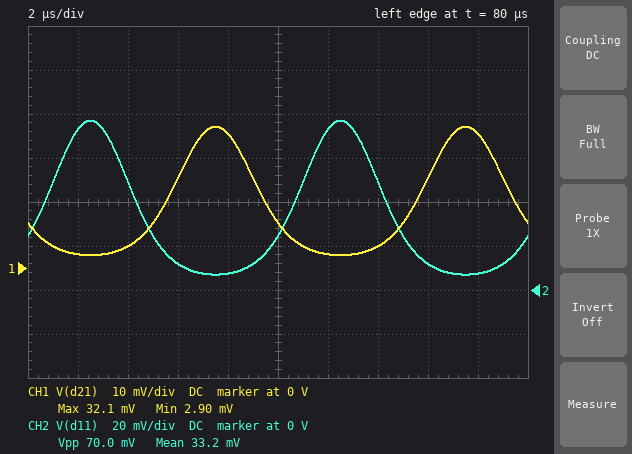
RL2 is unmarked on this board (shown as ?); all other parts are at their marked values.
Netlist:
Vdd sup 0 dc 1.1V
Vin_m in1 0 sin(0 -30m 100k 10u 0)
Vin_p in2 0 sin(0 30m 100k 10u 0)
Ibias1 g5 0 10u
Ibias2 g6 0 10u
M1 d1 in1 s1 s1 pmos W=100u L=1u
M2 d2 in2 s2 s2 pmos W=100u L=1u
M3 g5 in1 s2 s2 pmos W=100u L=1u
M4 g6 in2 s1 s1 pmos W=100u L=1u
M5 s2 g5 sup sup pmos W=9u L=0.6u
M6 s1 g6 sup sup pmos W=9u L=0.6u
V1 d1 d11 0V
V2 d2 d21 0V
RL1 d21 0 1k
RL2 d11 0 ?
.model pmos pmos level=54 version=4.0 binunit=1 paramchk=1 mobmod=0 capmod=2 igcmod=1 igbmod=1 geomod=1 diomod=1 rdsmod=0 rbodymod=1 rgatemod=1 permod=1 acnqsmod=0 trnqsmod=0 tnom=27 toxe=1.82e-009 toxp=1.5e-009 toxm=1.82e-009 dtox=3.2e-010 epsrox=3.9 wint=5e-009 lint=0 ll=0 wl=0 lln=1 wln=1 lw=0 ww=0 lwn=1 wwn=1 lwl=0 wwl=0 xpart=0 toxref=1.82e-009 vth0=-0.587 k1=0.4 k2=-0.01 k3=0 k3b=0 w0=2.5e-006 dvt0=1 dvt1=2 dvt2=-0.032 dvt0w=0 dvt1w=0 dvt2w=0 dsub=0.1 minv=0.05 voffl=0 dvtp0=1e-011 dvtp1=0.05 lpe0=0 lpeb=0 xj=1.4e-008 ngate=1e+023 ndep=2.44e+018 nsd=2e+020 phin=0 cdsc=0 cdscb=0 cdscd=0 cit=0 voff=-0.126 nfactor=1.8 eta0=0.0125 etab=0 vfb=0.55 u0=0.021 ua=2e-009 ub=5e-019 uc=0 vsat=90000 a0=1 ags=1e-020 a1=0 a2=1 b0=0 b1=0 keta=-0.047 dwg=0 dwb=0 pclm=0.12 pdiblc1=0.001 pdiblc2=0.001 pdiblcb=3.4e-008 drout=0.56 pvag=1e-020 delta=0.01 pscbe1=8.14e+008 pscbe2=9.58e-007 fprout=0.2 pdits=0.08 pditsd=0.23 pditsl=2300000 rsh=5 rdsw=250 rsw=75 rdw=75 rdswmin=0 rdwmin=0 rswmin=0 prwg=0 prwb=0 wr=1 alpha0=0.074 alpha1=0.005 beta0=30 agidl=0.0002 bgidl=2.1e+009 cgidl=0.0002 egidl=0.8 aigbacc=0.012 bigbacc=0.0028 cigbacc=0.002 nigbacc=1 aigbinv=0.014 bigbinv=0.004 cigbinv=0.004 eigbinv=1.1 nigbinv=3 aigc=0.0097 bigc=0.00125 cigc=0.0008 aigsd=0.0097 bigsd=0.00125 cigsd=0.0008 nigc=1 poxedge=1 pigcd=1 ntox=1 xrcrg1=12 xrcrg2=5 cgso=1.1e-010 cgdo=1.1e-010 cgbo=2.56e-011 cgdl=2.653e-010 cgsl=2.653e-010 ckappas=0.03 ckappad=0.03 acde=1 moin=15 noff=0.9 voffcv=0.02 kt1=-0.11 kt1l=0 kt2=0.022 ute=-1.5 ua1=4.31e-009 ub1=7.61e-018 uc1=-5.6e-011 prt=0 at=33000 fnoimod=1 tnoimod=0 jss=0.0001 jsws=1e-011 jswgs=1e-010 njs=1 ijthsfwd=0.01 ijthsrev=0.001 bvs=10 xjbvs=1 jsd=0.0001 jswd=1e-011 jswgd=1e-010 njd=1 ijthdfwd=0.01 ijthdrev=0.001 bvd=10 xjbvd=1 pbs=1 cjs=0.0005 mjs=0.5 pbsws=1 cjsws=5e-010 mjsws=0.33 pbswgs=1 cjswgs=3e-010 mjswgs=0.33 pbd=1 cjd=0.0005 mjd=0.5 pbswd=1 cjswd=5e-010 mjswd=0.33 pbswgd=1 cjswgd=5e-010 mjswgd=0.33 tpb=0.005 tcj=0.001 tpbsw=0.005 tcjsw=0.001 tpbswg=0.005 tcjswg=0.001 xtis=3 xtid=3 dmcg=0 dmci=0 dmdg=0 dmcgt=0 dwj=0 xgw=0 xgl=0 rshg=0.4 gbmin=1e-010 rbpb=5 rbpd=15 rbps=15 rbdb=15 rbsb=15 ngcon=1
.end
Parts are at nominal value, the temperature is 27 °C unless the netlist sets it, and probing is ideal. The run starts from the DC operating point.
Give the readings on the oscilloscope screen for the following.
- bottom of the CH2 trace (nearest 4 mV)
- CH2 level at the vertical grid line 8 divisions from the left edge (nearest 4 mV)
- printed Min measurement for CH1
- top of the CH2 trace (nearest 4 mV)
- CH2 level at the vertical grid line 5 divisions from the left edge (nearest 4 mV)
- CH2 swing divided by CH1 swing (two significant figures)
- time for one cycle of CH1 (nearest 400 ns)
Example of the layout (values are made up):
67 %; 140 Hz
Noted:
8 mV; 12 mV; 2.90 mV; 76 mV; 24 mV; 2.4; 10.0 µs
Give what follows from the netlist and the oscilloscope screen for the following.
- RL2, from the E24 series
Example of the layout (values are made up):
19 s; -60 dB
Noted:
2.4 kΩ
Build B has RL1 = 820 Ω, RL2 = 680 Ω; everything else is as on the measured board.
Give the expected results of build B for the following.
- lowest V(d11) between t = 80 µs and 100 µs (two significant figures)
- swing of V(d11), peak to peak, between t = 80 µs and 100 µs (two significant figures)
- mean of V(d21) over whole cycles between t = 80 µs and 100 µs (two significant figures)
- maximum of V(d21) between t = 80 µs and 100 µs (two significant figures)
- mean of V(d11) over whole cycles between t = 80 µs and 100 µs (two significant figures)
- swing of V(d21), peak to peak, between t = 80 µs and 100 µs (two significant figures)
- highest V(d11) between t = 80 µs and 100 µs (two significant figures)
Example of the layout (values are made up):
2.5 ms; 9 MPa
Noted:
2.0 mV; 20 mV; 11 mV; 26 mV; 9.4 mV; 24 mV; 22 mV
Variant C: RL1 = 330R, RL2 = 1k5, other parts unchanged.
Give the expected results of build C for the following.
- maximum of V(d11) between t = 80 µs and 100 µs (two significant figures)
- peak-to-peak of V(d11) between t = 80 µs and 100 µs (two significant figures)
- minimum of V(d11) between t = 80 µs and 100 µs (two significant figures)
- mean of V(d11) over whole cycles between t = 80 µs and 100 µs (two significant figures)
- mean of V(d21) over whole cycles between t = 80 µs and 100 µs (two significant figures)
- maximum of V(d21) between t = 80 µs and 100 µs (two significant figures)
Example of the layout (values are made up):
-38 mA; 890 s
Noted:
48 mV; 44 mV; 4.4 mV; 21 mV; 4.6 mV; 11 mV
